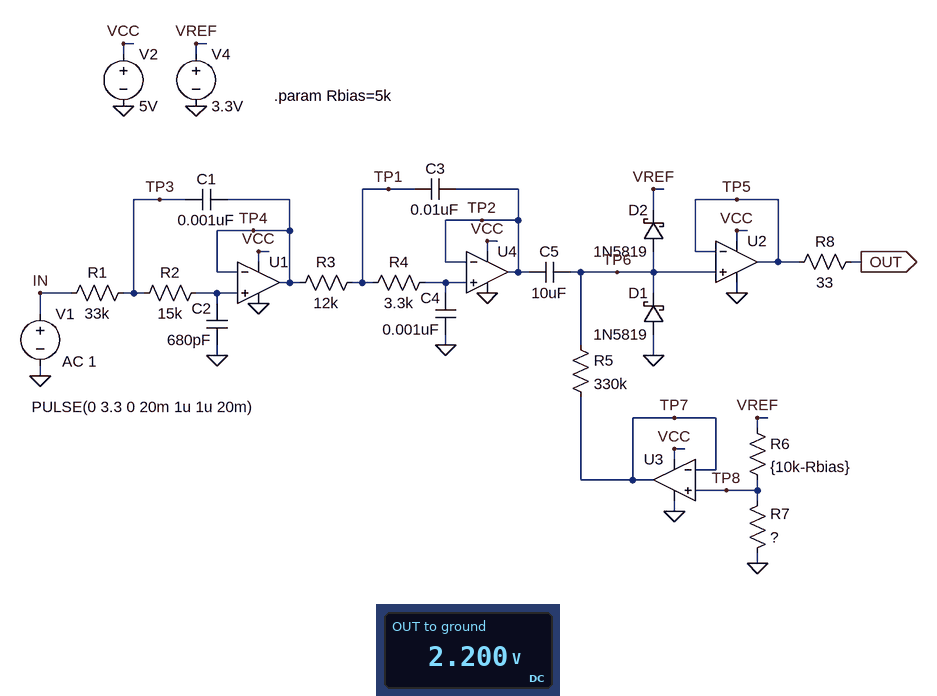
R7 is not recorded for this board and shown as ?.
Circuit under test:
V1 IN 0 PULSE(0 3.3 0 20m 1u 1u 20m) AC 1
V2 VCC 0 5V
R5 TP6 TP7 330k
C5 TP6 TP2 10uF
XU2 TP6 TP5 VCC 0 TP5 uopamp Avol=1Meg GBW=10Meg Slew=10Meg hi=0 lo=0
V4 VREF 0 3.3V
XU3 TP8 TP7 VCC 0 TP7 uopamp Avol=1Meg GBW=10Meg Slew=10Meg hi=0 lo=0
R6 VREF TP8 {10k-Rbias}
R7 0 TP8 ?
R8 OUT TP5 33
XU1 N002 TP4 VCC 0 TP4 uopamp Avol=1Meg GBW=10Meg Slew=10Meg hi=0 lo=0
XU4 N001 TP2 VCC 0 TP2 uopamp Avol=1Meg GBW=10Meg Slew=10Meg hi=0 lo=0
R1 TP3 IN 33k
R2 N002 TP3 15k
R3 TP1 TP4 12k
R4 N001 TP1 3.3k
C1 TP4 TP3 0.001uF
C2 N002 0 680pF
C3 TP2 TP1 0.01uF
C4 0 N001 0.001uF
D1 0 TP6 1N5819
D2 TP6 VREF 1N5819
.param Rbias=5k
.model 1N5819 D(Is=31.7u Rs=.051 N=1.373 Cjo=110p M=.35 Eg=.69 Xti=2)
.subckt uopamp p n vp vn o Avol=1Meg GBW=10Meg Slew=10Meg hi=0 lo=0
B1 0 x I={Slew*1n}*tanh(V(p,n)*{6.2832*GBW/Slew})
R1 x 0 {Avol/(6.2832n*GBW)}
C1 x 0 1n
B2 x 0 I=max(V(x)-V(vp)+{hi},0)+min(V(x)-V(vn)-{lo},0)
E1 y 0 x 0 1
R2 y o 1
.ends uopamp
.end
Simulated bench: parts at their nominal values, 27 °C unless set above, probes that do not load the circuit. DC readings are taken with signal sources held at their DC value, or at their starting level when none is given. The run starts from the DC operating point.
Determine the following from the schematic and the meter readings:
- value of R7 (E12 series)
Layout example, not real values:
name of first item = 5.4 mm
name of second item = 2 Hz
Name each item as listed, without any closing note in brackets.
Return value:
value of R7 = 10 kΩ
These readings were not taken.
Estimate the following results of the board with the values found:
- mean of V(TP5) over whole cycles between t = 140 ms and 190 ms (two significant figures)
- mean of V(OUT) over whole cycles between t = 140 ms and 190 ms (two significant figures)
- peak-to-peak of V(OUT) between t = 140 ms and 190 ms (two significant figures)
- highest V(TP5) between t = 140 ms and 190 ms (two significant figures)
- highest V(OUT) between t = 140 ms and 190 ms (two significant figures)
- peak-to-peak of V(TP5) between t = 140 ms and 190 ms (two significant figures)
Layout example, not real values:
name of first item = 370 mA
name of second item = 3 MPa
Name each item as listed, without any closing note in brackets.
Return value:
mean of V(TP5) over whole cycles between t = 140 ms and 190 ms = 1.7 V
mean of V(OUT) over whole cycles between t = 140 ms and 190 ms = 1.7 V
peak-to-peak of V(OUT) between t = 140 ms and 190 ms = 3.3 V
highest V(TP5) between t = 140 ms and 190 ms = 3.4 V
highest V(OUT) between t = 140 ms and 190 ms = 3.4 V
peak-to-peak of V(TP5) between t = 140 ms and 190 ms = 3.3 V
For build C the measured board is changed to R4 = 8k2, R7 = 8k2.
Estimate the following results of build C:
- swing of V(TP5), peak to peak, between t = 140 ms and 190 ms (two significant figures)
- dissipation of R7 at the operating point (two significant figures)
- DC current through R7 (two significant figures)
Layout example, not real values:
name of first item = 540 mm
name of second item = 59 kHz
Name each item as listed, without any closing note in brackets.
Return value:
swing of V(TP5), peak to peak, between t = 140 ms and 190 ms = 3.3 V
dissipation of R7 at the operating point = 510 µW
DC current through R7 = 250 µA
